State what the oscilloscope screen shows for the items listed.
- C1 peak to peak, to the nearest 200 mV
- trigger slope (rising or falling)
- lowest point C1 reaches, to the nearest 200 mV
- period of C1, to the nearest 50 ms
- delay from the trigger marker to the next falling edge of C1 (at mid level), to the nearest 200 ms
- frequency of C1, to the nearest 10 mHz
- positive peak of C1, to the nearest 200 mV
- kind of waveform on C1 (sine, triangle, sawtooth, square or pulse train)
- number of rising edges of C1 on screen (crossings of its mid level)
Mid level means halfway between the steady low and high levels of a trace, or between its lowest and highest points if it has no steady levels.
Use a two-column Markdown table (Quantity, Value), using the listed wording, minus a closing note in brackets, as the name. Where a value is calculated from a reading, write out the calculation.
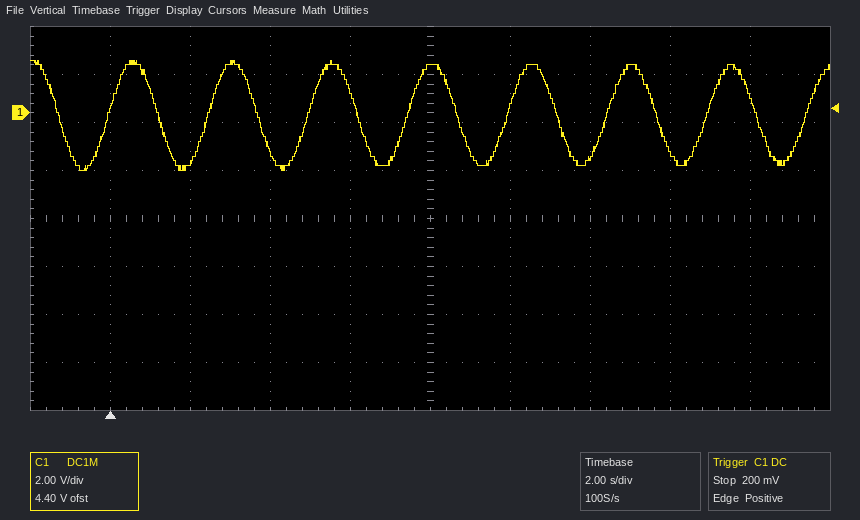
| Quantity | Value |
|---|---|
| C1 peak to peak, to the nearest 200 mV | 2.2 V − (-2.4 V) = 4.6 V |
| trigger slope | rising |
| lowest point C1 reaches, to the nearest 200 mV | -2.4 V |
| period of C1, to the nearest 50 ms | 2.50 s |
| delay from the trigger marker to the next falling edge of C1 (at mid level), to the nearest 200 ms | 1.2 s |
| frequency of C1, to the nearest 10 mHz | 1 / 2.50 s ≈ 400 mHz |
| positive peak of C1, to the nearest 200 mV | 2.2 V |
| kind of waveform on C1 | sine |
| number of rising edges of C1 on screen | 8 |
